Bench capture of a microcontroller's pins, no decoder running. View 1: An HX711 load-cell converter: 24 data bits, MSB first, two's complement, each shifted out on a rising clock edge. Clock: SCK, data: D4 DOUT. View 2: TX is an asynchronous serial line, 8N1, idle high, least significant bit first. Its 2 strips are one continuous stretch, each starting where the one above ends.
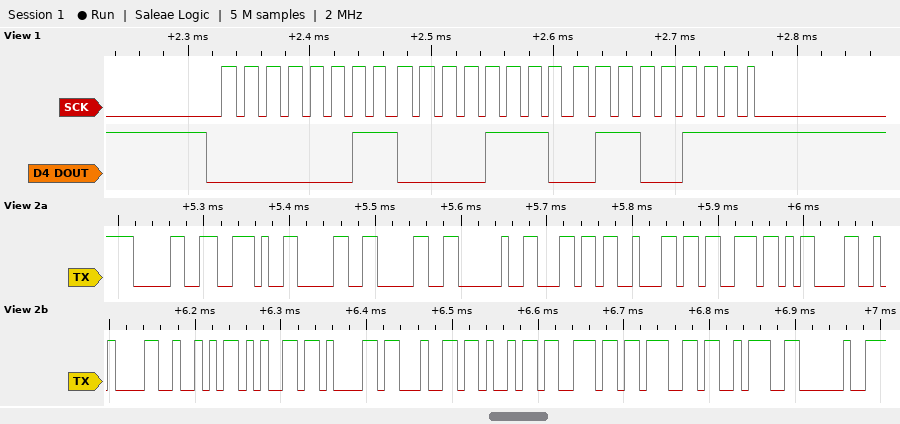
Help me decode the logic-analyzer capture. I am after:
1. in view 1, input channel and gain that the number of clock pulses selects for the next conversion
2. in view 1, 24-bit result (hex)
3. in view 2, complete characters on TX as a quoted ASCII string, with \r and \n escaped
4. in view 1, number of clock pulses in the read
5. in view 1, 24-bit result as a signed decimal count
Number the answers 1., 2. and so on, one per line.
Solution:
1. channel A, gain 128
2. 0x030E67
3. "0.00 lbs\r\nReading: "
4. 25
5. 200295
